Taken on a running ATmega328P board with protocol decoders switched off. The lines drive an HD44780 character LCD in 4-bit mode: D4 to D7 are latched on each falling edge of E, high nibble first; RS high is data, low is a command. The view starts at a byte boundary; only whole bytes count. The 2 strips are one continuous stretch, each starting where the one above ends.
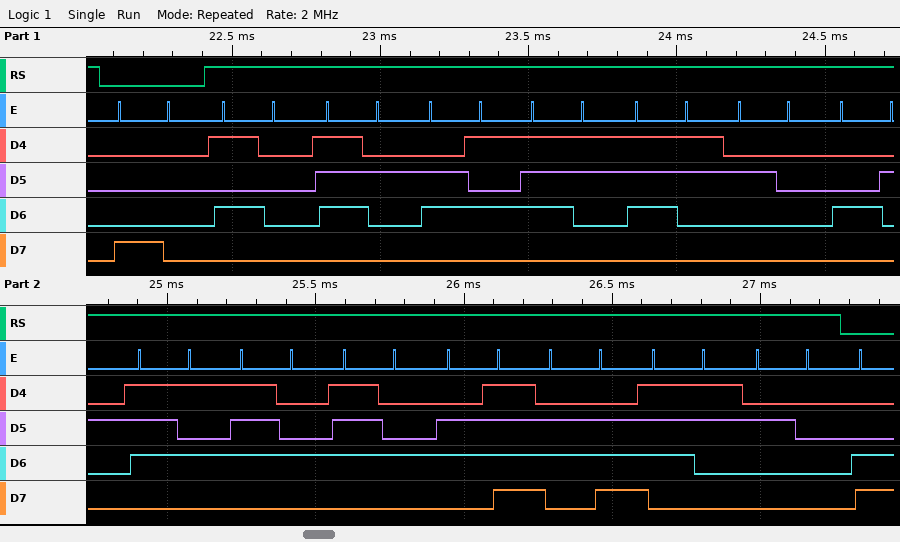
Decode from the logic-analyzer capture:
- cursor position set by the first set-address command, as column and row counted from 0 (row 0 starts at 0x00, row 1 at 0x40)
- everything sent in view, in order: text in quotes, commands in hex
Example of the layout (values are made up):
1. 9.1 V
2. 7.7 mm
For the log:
1. column 0, row 0
2. 0x80 "Press Buttons "
